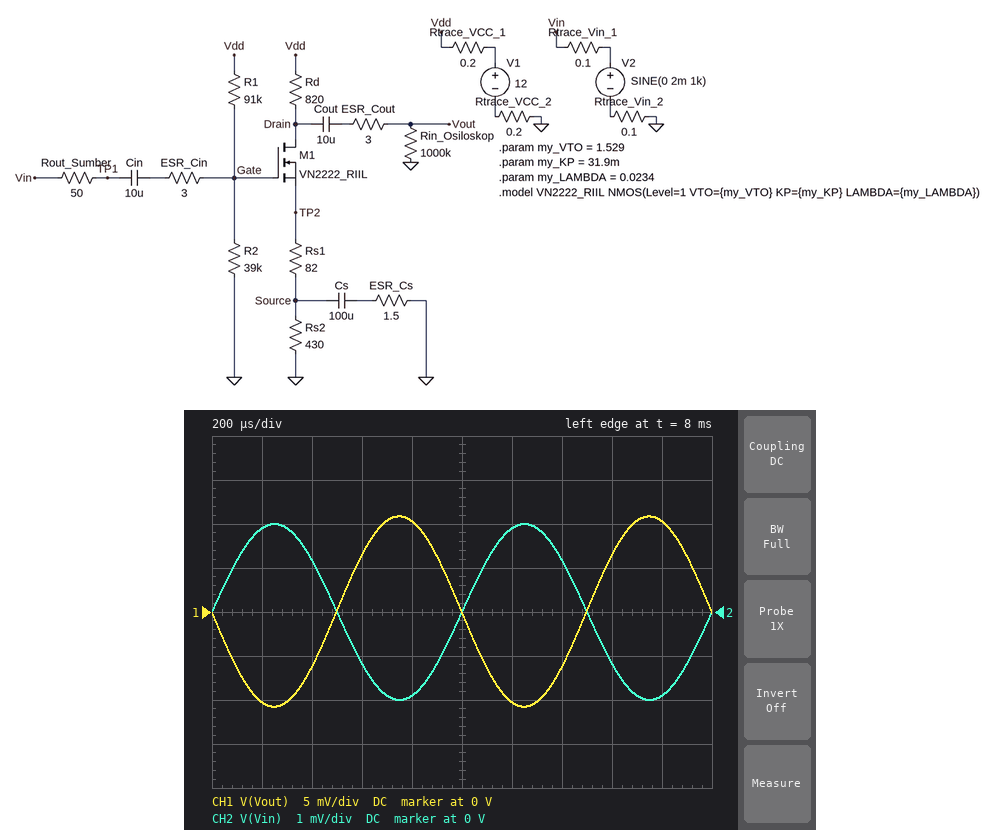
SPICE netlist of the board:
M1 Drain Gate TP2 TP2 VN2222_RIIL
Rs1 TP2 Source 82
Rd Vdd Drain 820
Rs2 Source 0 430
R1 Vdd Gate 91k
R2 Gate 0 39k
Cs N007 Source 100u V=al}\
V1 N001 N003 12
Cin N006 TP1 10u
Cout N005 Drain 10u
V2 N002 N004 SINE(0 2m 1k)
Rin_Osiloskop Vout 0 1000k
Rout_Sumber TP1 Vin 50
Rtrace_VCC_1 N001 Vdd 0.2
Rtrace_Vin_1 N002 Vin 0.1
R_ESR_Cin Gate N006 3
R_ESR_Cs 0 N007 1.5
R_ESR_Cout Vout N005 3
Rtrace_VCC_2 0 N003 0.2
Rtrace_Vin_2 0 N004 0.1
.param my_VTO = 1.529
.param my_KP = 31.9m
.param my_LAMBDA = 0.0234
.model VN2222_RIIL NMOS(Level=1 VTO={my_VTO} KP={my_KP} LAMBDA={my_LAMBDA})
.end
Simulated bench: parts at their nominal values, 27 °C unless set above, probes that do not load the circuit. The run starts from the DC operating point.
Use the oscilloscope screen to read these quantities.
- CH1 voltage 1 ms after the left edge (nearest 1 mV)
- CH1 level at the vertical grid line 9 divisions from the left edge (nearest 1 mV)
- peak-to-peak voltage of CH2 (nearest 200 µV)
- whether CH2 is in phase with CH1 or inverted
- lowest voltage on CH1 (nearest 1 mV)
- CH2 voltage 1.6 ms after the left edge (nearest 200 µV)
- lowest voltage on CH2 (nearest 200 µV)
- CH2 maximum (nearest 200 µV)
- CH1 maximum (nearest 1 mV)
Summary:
0 V
10 mV
4.0 mV
inverted
-11 mV
-1.2 mV
-2.0 mV
2.0 mV
11 mV
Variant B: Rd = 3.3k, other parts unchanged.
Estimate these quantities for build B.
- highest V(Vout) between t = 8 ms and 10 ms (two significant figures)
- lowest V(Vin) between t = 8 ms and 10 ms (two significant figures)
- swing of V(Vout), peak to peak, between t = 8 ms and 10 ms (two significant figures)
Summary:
2.1 mV
-2.0 mV
4.2 mV
